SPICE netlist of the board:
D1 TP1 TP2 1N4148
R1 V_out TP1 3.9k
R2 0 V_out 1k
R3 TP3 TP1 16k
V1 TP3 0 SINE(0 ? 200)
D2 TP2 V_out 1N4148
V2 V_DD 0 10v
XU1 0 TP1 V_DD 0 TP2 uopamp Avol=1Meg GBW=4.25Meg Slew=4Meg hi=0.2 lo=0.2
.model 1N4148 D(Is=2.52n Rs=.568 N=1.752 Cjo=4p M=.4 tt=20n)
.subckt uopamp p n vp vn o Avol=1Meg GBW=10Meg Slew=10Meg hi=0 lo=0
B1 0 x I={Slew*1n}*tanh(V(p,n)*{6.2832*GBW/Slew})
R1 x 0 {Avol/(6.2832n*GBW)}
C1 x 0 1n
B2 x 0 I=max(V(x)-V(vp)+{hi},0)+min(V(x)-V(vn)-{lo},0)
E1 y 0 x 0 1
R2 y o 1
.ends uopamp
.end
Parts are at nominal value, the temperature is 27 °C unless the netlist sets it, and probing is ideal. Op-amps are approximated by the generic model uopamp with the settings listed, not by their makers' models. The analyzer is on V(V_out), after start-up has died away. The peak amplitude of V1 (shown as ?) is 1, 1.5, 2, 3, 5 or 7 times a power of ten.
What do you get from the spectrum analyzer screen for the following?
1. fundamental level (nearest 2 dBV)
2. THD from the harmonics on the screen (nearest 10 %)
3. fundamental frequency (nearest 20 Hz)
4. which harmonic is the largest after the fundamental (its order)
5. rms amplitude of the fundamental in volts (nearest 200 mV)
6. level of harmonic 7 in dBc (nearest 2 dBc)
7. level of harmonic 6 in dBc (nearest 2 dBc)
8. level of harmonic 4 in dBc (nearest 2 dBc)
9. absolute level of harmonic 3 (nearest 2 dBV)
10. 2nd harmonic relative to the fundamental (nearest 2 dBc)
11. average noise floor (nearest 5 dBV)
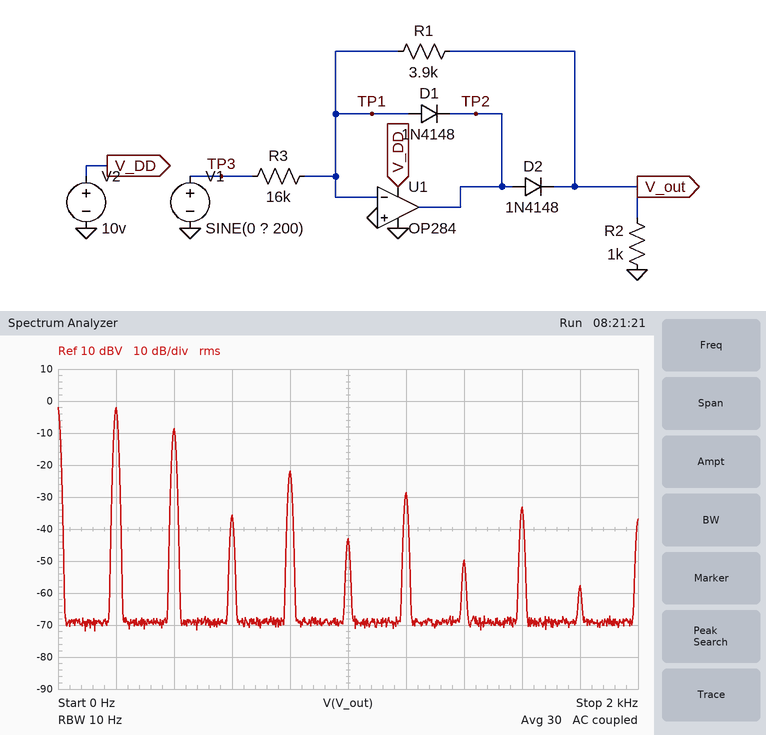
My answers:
-2 dBV
50 %
200 Hz
2
800 mV
-48 dBc
-26 dBc
-20 dBc
-36 dBV
-6 dBc
-70 dBV
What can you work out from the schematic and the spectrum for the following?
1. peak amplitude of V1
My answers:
10 V
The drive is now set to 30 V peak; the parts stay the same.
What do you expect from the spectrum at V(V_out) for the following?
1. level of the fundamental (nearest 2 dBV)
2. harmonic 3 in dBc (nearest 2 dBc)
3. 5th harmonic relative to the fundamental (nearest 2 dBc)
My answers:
8 dBV
-42 dBc
-46 dBc
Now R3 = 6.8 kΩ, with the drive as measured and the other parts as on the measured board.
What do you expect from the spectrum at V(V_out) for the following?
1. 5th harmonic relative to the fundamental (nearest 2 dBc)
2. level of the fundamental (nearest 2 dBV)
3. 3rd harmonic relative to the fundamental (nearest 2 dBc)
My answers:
-46 dBc
6 dBV
-40 dBc
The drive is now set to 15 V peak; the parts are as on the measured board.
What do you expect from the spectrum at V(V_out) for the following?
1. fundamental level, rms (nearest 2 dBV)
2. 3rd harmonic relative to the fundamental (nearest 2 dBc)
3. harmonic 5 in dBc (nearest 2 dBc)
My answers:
2 dBV
-36 dBc
-42 dBc
